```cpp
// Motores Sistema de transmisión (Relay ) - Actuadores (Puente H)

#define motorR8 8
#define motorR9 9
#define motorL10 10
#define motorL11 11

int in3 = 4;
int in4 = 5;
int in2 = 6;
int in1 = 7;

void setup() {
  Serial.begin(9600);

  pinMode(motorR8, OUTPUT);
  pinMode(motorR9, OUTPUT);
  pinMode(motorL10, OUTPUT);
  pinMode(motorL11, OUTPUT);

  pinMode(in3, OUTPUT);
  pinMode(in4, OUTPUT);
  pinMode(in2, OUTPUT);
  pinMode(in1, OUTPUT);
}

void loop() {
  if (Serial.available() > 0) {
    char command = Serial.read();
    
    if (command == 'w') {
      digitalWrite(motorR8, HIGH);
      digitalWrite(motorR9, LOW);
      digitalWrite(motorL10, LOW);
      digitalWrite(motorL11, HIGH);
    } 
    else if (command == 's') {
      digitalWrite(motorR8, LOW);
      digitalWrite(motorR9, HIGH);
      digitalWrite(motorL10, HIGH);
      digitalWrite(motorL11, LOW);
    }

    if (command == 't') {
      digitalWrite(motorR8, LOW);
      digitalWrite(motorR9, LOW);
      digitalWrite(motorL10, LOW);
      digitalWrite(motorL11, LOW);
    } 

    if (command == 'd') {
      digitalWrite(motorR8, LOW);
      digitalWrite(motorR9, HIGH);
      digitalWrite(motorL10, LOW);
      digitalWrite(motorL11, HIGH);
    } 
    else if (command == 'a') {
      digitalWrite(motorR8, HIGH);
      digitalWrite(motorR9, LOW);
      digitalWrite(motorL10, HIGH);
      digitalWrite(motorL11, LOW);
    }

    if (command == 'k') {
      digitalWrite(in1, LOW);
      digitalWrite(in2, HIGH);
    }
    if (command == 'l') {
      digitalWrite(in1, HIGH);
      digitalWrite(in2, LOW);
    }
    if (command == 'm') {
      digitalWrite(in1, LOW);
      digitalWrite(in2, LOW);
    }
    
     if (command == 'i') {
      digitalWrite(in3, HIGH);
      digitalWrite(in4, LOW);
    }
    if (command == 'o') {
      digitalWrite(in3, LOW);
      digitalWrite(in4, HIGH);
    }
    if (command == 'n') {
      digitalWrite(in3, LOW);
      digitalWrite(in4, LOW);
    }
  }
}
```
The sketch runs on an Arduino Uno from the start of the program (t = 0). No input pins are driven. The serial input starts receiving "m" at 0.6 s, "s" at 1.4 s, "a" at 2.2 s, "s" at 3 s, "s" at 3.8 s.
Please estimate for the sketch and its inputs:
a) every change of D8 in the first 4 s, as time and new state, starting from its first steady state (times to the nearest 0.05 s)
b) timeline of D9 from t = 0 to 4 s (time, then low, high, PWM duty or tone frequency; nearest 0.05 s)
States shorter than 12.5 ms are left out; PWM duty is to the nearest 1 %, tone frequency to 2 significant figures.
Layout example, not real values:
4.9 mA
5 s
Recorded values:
0 s low; 2.2 s high; 3 s low
0 s low; 1.4 s high; 2.2 s low; 3 s high
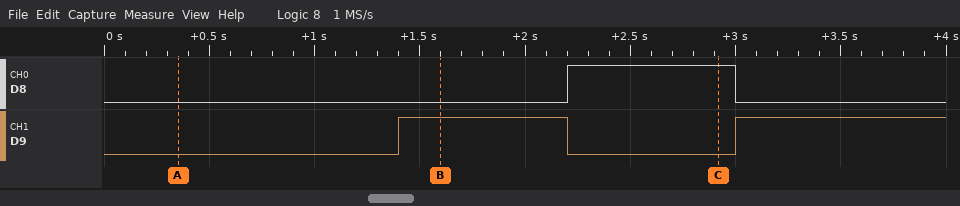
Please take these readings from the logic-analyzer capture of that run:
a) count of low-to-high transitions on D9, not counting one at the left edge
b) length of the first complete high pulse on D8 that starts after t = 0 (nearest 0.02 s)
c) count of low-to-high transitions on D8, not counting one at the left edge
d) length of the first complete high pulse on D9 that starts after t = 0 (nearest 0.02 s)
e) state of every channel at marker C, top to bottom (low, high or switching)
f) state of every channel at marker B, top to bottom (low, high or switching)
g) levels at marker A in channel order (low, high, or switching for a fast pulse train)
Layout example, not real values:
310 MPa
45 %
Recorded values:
2
0.80 s
1
0.80 s
D8 high, D9 low
D8 low, D9 high
D8 low, D9 low
